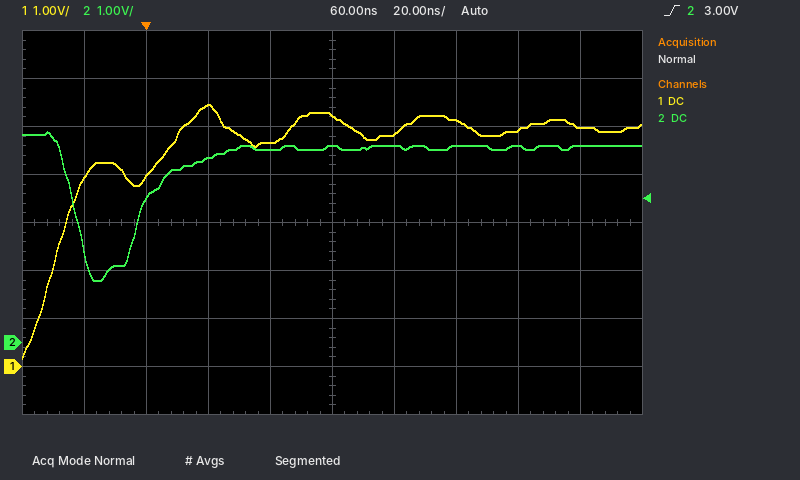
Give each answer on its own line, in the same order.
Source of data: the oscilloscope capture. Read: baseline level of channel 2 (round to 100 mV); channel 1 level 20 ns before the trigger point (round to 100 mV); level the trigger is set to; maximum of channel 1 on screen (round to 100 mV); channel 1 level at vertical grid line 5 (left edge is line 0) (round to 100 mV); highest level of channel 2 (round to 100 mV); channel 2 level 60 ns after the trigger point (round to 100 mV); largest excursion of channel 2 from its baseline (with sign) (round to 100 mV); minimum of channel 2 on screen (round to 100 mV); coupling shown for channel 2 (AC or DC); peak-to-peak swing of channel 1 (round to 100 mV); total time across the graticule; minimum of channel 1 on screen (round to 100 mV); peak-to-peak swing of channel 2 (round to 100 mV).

4.1 V
3.9 V
3.00 V
5.5 V
5.2 V
4.4 V
4.1 V
-2.8 V
1.3 V
DC
5.3 V
200 ns
200 mV
3.1 V
